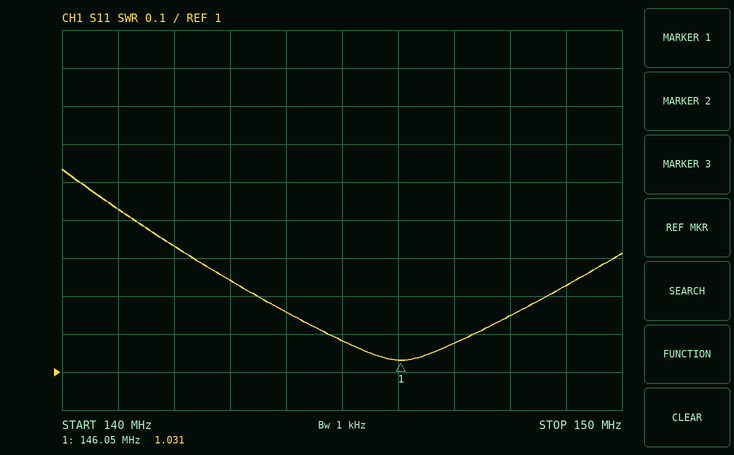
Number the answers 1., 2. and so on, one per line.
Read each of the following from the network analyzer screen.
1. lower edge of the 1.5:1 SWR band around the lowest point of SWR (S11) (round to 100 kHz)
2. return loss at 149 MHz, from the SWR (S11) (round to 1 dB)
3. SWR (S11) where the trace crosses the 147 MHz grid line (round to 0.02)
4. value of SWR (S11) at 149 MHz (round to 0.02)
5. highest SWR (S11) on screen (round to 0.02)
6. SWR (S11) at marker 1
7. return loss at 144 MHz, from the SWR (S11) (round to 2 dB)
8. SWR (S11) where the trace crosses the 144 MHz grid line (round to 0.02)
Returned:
1. 140.3 MHz
2. 20 dB
3. 1.08
4. 1.22
5. 1.54
6. 1.031
7. 22 dB
8. 1.16
